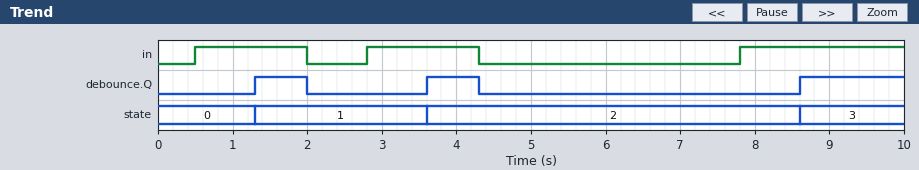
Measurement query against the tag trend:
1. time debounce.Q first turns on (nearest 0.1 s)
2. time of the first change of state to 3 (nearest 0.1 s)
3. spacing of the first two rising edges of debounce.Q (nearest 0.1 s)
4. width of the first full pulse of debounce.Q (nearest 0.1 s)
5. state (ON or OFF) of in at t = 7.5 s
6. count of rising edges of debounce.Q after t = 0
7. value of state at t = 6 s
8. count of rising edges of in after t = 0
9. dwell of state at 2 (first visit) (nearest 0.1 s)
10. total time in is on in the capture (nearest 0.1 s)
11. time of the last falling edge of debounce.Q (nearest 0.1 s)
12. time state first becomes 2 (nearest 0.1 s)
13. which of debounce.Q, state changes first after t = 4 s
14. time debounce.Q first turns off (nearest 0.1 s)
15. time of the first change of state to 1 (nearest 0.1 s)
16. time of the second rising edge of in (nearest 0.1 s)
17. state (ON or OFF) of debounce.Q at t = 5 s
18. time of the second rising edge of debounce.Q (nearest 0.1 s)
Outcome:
1.3 s
8.6 s
2.3 s
0.7 s
OFF
3
2
3
5.0 s
5.2 s
4.3 s
3.6 s
debounce.Q
2.0 s
1.3 s
2.8 s
OFF
3.6 s
